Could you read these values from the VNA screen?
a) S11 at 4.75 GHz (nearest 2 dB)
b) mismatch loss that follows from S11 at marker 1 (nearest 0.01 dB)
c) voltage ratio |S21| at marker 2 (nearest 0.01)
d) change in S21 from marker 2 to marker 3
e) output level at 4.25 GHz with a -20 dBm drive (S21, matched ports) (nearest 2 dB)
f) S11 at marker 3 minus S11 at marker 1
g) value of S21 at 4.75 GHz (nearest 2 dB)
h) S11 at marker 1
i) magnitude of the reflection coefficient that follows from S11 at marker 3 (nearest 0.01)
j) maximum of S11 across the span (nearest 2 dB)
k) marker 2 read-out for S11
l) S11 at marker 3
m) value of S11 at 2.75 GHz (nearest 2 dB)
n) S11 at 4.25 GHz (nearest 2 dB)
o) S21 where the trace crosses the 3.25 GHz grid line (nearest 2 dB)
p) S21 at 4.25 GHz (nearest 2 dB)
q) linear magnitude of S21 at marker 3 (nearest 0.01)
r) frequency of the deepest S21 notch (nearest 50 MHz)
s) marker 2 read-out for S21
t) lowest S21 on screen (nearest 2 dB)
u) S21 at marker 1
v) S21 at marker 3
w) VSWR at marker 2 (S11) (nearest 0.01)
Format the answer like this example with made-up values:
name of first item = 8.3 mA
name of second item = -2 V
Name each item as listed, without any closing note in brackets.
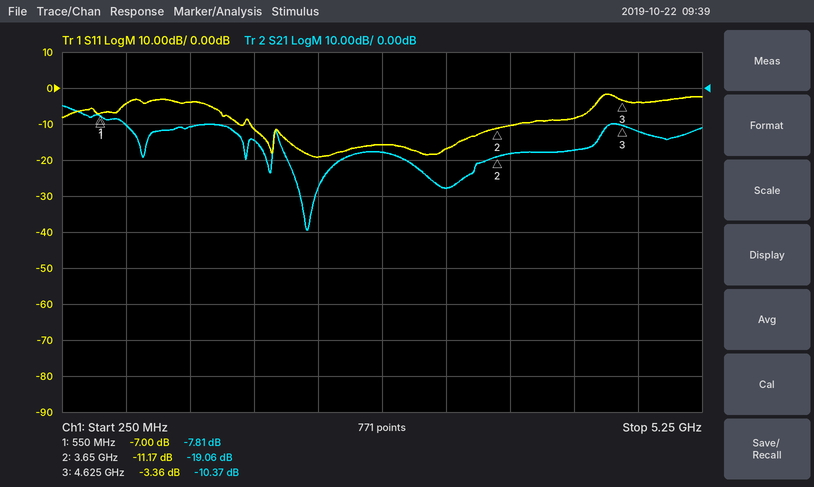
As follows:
S11 at 4.75 GHz = -4 dB
mismatch loss that follows from S11 at marker 1 = 0.97 dB
voltage ratio |S21| at marker 2 = 0.11
change in S21 from marker 2 to marker 3 = 8.69 dB
output level at 4.25 GHz with a -20 dBm drive (S21, matched ports) = -38 dBm
S11 at marker 3 minus S11 at marker 1 = 3.64 dB
value of S21 at 4.75 GHz = -12 dB
S11 at marker 1 = -7.00 dB
magnitude of the reflection coefficient that follows from S11 at marker 3 = 0.68
maximum of S11 across the span = -2 dB
marker 2 read-out for S11 = -11.17 dB
S11 at marker 3 = -3.36 dB
value of S11 at 2.75 GHz = -16 dB
S11 at 4.25 GHz = -8 dB
S21 where the trace crosses the 3.25 GHz grid line = -28 dB
S21 at 4.25 GHz = -18 dB
linear magnitude of S21 at marker 3 = 0.30
frequency of the deepest S21 notch = 2.15 GHz
marker 2 read-out for S21 = -19.06 dB
lowest S21 on screen = -40 dB
S21 at marker 1 = -7.81 dB
S21 at marker 3 = -10.37 dB
VSWR at marker 2 (S11) = 1.76
